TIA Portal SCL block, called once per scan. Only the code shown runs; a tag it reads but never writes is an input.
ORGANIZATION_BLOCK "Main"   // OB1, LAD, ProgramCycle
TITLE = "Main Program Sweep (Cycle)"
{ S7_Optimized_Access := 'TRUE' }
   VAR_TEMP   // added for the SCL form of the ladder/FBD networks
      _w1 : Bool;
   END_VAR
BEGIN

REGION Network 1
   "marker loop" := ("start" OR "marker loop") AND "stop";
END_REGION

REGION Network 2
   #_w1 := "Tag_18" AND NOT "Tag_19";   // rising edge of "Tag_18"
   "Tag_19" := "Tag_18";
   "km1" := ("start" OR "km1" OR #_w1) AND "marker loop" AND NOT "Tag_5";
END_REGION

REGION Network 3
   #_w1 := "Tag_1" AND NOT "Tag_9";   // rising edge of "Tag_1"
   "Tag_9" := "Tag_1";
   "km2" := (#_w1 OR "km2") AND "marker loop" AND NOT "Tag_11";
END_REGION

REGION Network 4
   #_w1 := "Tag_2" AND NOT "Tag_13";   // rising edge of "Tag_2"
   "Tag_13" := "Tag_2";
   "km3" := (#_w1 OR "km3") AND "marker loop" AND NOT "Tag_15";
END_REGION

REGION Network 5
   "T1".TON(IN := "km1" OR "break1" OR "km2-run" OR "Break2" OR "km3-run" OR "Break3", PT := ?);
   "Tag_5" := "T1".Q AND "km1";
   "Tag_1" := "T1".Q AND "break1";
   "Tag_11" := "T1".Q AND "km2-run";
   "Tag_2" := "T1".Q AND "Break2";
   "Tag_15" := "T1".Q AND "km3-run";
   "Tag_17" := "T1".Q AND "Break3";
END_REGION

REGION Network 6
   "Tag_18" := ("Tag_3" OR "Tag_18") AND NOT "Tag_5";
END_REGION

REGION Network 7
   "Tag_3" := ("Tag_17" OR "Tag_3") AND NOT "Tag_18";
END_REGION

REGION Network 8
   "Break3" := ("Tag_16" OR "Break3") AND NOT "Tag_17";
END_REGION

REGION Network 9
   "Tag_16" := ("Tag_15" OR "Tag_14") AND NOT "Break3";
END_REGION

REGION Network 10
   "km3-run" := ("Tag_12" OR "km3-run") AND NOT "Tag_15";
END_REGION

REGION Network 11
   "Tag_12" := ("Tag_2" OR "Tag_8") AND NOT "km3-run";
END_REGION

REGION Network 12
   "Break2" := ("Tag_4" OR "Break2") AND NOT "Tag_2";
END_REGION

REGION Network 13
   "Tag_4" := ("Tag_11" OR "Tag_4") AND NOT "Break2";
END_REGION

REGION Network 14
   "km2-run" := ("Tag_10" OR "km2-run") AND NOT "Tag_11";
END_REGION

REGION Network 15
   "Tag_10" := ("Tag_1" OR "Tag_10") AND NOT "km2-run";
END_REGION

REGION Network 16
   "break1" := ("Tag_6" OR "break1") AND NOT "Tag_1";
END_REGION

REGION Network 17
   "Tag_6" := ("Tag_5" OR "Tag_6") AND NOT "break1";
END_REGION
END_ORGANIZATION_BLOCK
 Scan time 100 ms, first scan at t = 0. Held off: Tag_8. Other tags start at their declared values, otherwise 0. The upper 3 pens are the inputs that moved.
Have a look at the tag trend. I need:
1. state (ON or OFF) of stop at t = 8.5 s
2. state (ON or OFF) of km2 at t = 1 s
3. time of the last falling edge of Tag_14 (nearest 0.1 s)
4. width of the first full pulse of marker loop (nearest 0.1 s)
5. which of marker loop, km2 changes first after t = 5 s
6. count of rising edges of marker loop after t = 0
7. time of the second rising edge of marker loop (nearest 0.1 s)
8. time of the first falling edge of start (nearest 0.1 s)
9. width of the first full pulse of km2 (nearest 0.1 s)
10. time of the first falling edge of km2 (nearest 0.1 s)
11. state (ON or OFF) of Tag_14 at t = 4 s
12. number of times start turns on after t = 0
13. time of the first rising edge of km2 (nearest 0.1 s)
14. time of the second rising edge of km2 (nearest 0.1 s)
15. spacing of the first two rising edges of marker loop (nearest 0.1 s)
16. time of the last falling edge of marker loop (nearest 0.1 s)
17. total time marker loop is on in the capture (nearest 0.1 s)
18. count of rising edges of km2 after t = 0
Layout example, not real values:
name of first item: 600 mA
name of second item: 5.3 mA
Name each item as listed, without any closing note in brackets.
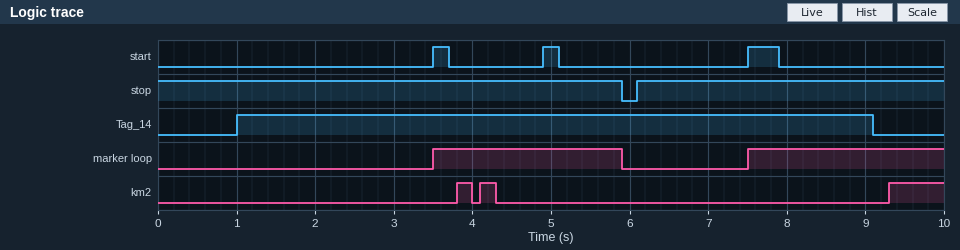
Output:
state (ON or OFF) of stop at t = 8.5 s: ON
state (ON or OFF) of km2 at t = 1 s: OFF
time of the last falling edge of Tag_14: 9.1 s
width of the first full pulse of marker loop: 2.4 s
which of marker loop, km2 changes first after t = 5 s: marker loop
count of rising edges of marker loop after t = 0: 2
time of the second rising edge of marker loop: 7.5 s
time of the first falling edge of start: 3.7 s
width of the first full pulse of km2: 0.2 s
time of the first falling edge of km2: 4.0 s
state (ON or OFF) of Tag_14 at t = 4 s: ON
number of times start turns on after t = 0: 3
time of the first rising edge of km2: 3.8 s
time of the second rising edge of km2: 4.1 s
spacing of the first two rising edges of marker loop: 4.0 s
time of the last falling edge of marker loop: 5.9 s
total time marker loop is on in the capture: 4.9 s
count of rising edges of km2 after t = 0: 3
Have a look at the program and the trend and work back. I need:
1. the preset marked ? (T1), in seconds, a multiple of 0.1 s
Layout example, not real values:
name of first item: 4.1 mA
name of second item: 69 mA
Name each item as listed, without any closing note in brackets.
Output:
the preset marked ? (T1), in seconds, a multiple of 0.1 s: 1.0 s
